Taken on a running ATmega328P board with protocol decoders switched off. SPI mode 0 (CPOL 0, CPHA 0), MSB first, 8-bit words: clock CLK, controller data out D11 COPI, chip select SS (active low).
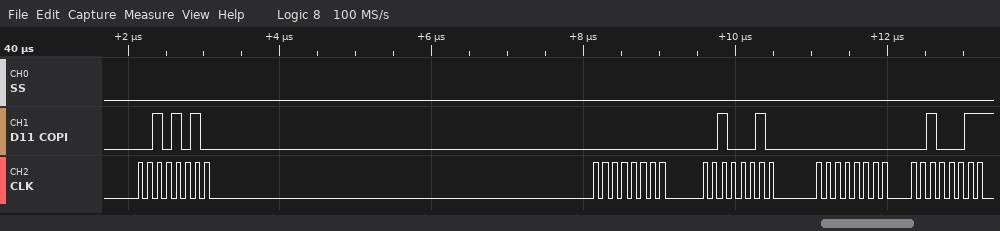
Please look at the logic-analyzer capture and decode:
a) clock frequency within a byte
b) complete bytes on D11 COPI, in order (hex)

8 MHz
2A 00 22 00 23
